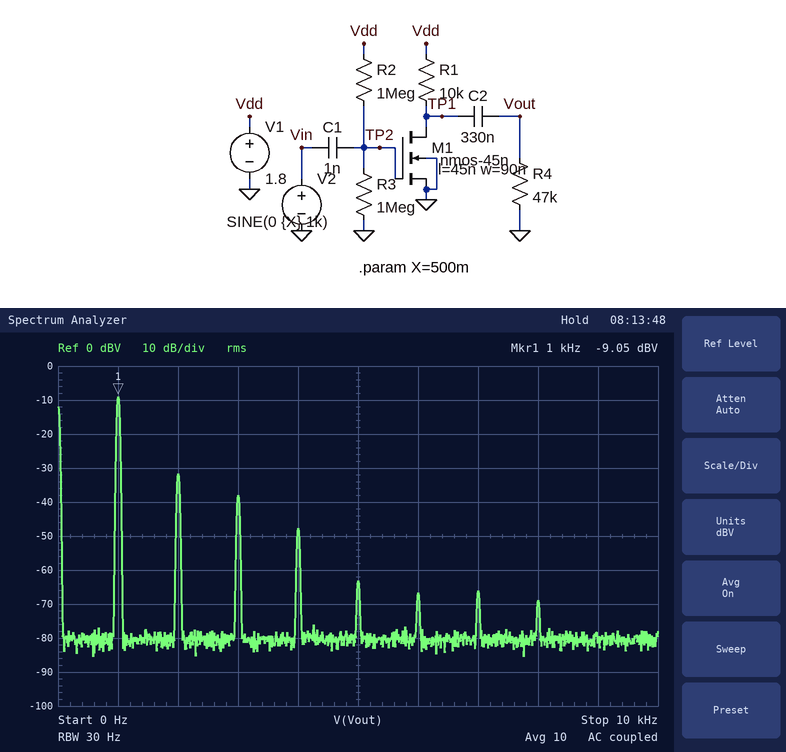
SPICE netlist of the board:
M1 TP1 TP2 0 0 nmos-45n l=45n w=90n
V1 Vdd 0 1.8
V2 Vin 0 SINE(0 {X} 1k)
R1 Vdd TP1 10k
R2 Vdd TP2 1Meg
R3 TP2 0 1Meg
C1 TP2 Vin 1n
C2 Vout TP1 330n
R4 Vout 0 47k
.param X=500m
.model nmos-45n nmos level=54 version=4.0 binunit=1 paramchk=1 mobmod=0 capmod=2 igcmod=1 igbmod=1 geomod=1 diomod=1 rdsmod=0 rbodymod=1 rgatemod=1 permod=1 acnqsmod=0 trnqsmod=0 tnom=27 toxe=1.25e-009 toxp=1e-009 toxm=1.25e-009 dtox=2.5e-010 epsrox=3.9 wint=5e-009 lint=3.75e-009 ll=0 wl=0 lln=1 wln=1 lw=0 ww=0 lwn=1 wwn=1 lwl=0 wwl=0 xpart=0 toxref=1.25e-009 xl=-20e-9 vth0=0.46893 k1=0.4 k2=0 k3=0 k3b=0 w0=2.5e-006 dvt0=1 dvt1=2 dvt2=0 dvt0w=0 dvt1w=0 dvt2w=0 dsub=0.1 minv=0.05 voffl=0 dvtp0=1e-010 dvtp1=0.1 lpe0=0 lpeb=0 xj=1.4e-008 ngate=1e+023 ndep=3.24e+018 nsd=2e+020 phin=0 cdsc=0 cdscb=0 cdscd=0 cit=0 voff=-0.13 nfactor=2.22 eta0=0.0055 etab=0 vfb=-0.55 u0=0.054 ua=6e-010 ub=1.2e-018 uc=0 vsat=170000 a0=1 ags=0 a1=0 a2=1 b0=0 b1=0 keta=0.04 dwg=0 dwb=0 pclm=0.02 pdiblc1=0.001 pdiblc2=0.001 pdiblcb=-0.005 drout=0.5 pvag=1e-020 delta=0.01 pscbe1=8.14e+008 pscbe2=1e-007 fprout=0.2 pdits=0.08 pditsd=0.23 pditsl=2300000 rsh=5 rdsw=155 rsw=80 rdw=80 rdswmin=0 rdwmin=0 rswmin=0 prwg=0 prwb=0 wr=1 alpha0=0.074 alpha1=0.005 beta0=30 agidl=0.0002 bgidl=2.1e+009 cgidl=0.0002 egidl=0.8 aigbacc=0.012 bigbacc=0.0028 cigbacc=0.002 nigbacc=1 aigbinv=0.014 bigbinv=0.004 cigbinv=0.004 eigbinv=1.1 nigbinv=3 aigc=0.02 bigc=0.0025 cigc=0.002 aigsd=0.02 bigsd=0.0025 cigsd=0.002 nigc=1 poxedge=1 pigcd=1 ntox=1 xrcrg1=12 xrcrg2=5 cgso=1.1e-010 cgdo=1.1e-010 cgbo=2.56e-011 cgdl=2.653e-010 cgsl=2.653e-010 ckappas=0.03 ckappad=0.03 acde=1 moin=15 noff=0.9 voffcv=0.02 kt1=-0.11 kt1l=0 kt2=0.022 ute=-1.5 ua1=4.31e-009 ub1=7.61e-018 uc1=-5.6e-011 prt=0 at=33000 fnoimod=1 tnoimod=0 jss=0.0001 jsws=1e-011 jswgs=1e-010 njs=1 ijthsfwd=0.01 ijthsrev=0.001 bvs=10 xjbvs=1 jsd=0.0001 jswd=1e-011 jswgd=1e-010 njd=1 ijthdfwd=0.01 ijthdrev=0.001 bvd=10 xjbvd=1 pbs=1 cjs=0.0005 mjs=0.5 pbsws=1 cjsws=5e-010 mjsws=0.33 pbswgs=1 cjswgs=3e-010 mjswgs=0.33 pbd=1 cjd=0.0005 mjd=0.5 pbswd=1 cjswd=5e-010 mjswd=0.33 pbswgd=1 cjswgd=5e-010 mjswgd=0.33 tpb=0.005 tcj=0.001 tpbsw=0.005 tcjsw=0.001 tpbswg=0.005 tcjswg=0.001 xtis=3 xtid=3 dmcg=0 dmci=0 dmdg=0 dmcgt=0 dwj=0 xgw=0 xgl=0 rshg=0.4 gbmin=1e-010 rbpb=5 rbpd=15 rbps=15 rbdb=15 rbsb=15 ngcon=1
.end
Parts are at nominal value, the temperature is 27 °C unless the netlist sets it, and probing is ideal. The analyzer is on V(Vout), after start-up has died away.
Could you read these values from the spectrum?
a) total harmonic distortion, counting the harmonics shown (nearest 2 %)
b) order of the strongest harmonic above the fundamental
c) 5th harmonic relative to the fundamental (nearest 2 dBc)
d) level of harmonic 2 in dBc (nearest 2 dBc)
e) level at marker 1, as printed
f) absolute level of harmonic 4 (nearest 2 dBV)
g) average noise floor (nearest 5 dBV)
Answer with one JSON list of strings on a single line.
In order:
["8 %", "2", "-54 dBc", "-22 dBc", "-9.05 dBV", "-48 dBV", "-80 dBV"]
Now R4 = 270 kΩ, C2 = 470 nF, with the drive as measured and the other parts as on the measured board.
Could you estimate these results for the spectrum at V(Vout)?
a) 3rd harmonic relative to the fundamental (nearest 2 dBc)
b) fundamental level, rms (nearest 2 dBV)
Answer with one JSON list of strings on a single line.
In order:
["-28 dBc", "-8 dBV"]
